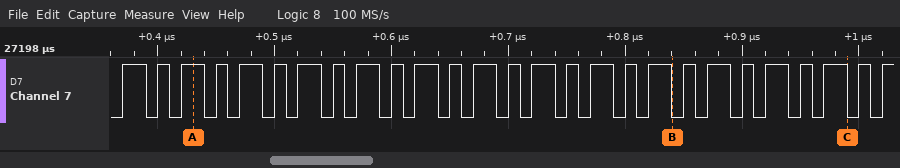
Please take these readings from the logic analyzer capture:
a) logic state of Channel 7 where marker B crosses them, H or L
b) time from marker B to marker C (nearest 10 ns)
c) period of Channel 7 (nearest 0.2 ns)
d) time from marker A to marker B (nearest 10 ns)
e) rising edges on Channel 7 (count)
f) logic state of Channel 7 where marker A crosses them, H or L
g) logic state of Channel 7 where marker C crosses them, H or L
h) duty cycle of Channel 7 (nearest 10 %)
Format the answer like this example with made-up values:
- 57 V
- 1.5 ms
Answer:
- Channel 7=L
- 150 ns
- 25 ns
- 410 ns
- 27
- Channel 7=H
- Channel 7=L
- 60 %
